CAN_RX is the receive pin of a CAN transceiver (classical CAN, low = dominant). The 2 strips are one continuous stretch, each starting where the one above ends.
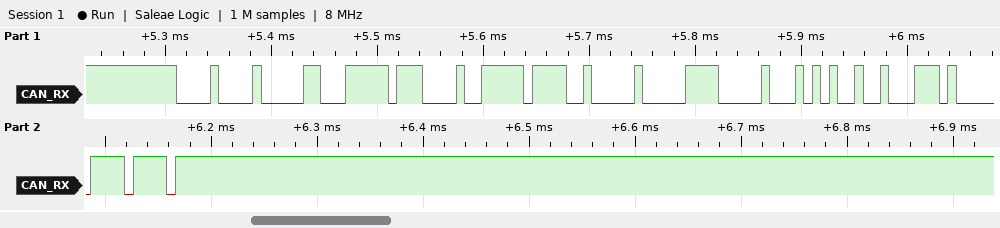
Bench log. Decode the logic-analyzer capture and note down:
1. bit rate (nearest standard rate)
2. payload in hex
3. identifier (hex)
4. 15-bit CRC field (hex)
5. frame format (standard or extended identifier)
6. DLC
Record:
125 kbit/s
FF 09 FF 20 07 00 A9 23
0x084
0x5077
standard
8
